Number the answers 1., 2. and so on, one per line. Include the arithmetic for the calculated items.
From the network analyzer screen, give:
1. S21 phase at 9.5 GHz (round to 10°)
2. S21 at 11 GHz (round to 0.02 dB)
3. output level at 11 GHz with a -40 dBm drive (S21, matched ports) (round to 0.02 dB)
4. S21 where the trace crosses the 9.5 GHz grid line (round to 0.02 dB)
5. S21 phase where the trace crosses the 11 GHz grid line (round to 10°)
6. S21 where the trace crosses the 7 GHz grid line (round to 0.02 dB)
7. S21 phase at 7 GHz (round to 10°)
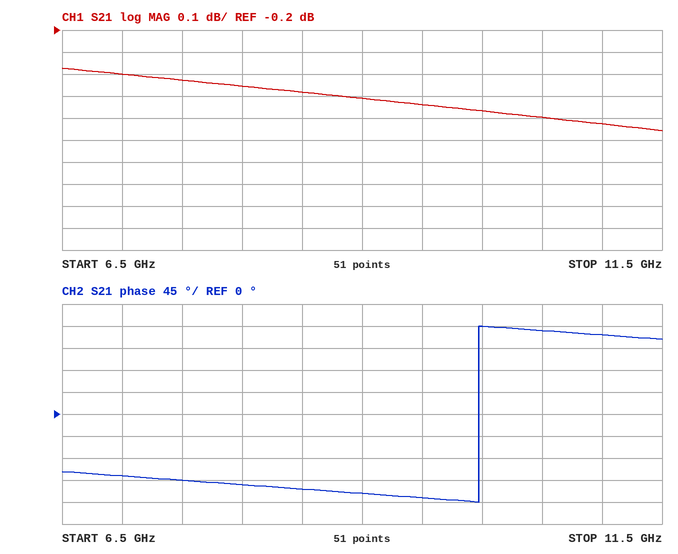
1. -170°
2. -0.62 dB
3. -40 dBm + (-0.62 dB) = -40.62 dBm
4. -0.54 dB
5. 160°
6. -0.40 dB
7. -130°
